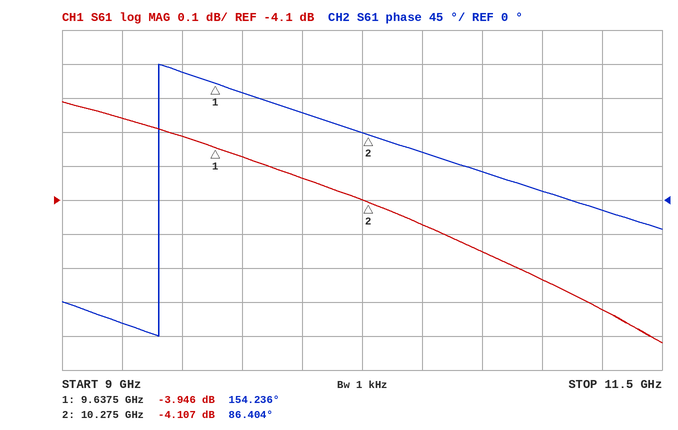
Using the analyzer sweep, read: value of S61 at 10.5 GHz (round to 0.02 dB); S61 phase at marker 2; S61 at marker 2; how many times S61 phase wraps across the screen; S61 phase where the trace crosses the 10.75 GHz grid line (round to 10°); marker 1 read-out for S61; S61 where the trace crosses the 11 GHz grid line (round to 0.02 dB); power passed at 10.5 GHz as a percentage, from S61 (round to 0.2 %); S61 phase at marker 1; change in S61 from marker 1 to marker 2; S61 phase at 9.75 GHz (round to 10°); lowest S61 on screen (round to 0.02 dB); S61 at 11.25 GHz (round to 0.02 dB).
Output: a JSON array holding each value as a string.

["-4.18 dB", "86.404°", "-4.107 dB", "1", "40°", "-3.946 dB", "-4.34 dB", "38.2 %", "154.236°", "-0.161 dB", "140°", "-4.52 dB", "-4.42 dB"]
